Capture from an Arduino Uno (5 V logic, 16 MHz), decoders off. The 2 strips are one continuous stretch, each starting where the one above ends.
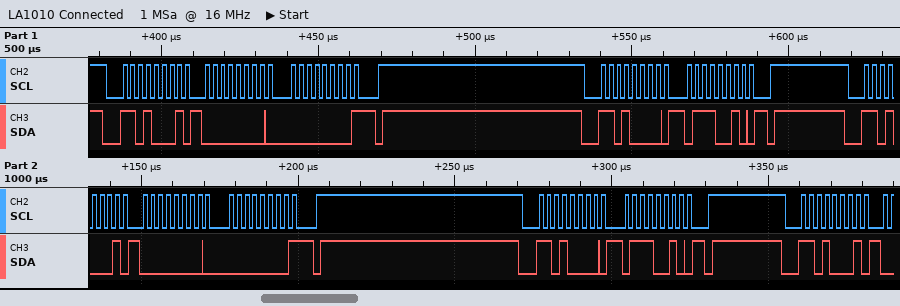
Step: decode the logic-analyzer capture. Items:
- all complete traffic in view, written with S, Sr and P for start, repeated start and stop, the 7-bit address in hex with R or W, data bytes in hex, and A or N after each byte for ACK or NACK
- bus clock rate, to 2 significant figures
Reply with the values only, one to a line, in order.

S 68R A 00 A 00 N P S 68W A 72 A P S 68R A 00 A 00 N P S 68W A 72 A P S 68R A
400 kHz
